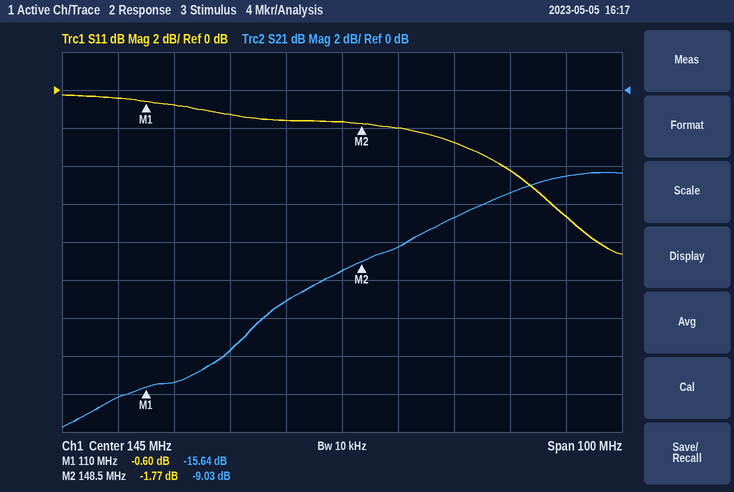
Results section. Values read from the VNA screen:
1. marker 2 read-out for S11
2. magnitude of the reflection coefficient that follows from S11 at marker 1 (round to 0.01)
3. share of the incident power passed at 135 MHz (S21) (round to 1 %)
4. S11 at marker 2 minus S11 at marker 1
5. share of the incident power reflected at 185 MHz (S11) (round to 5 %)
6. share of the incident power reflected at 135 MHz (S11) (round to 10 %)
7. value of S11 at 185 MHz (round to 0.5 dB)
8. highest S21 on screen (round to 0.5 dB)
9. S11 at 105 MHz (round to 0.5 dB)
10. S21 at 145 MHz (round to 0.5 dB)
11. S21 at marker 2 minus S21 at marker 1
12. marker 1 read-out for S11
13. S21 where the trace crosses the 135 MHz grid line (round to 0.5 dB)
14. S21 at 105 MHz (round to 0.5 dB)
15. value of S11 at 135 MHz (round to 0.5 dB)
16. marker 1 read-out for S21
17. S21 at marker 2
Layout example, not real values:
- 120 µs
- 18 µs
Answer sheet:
- -1.77 dB
- 0.93
- 8 %
- -1.17 dB
- 20 %
- 70 %
- -6.5 dB
- -4.5 dB
- -0.5 dB
- -9.5 dB
- 6.61 dB
- -0.60 dB
- -11.0 dB
- -16.0 dB
- -1.5 dB
- -15.64 dB
- -9.03 dB
